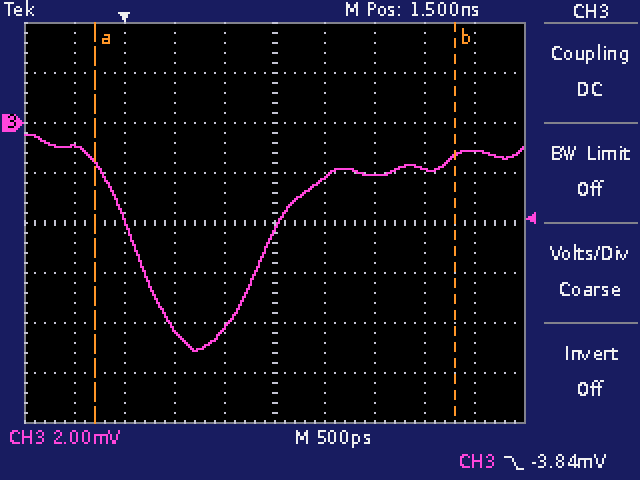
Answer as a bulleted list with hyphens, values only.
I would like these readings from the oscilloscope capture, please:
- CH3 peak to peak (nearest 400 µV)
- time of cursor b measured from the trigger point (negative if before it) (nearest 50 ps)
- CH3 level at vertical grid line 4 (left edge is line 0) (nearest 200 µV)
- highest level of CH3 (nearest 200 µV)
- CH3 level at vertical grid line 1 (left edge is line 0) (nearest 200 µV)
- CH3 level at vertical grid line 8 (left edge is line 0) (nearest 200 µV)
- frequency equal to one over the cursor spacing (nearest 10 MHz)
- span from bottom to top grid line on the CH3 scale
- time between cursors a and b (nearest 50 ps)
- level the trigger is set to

- 8.8 mV
- +3.30 ns
- -8.2 mV
- -400 µV
- -1.0 mV
- -1.8 mV
- 280 MHz
- 16 mV
- 3.60 ns
- -3.84 mV
